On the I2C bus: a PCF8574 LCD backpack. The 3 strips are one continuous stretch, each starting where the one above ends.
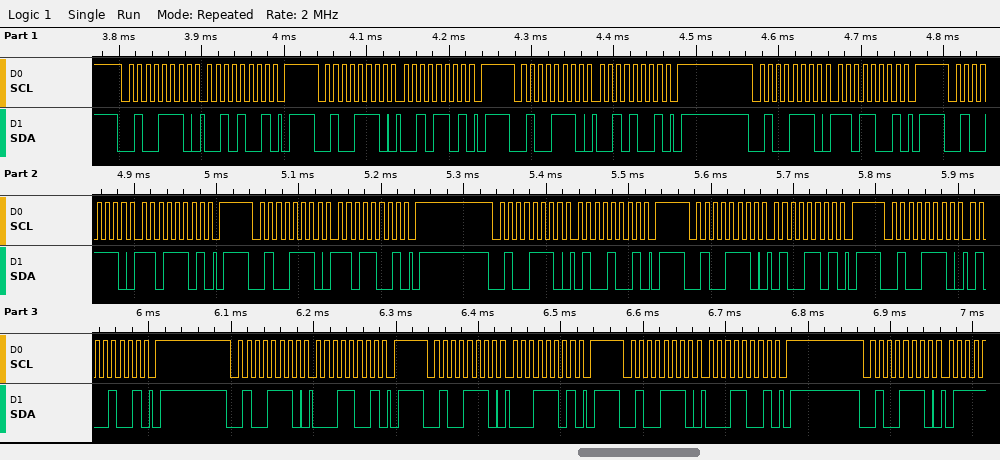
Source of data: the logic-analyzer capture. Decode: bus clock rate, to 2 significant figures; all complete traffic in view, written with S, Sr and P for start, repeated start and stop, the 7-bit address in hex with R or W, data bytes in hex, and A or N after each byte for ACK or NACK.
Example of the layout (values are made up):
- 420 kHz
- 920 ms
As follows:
- 100 kHz
- S 27W A 29 A P S 27W A 2D A P S 27W A 29 A P S 27W A D9 A P S 27W A DD A P S 27W A D9 A P S 27W A 49 A P S 27W A 4D A P S 27W A 49 A P S 27W A 19 A P S 27W A 1D A P S 27W A 19 A P S 27W A
